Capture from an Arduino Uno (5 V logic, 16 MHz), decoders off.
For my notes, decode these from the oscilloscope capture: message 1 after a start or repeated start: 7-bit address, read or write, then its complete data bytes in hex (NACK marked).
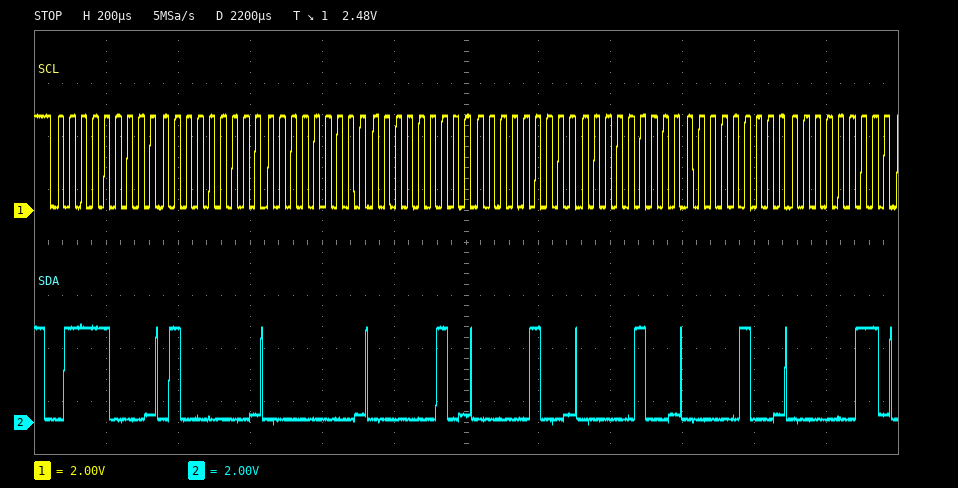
0x3C write: 40 00 02 04 04 04 03
